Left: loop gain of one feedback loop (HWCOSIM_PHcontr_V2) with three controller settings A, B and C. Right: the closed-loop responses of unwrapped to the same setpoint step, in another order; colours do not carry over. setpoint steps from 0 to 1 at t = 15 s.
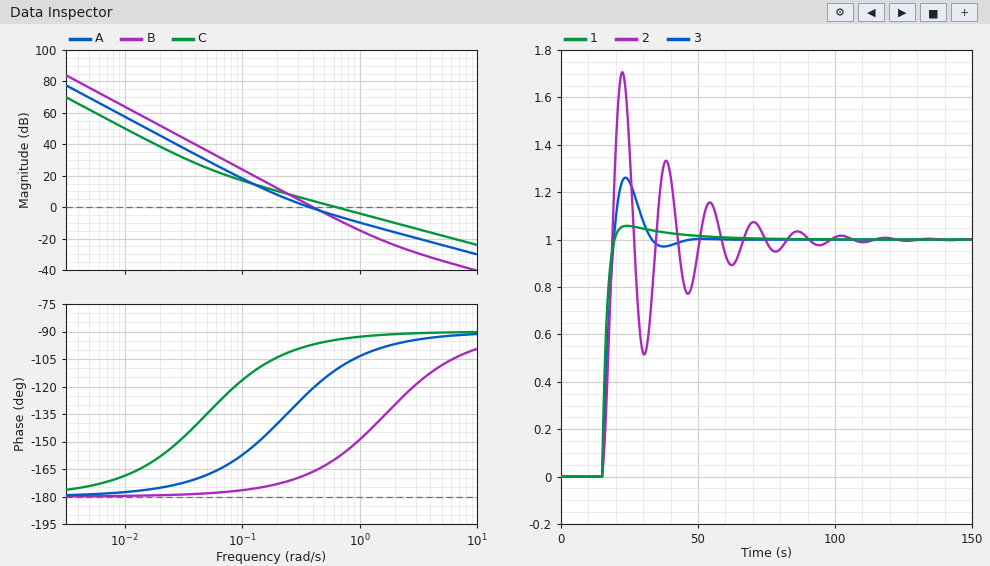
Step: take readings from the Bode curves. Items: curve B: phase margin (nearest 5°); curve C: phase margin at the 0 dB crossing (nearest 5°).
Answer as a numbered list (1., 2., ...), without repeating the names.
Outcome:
1. 15°
2. 85°
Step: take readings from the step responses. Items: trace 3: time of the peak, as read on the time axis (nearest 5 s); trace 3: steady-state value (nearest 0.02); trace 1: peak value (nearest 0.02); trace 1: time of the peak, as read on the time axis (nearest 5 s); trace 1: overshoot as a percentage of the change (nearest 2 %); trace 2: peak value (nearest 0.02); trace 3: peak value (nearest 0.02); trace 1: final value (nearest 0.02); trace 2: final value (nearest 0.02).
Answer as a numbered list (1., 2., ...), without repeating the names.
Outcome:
1. 25 s
2. 1.00
3. 1.06
4. 25 s
5. 6 %
6. 1.70
7. 1.26
8. 1.00
9. 1.00
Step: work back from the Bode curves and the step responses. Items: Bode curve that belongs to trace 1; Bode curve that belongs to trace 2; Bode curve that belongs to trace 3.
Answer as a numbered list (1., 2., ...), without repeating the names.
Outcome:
1. C
2. B
3. A
